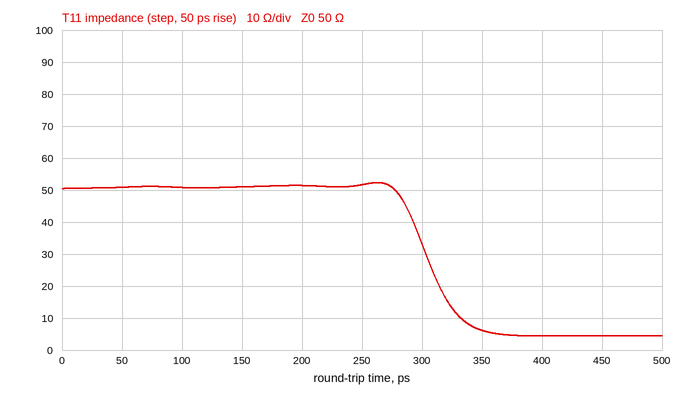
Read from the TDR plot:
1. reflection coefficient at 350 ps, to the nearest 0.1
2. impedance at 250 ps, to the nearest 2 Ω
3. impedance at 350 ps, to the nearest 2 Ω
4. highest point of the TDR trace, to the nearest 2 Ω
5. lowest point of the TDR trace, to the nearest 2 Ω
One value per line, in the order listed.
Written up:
-0.8
52 Ω
6 Ω
52 Ω
4 Ω
